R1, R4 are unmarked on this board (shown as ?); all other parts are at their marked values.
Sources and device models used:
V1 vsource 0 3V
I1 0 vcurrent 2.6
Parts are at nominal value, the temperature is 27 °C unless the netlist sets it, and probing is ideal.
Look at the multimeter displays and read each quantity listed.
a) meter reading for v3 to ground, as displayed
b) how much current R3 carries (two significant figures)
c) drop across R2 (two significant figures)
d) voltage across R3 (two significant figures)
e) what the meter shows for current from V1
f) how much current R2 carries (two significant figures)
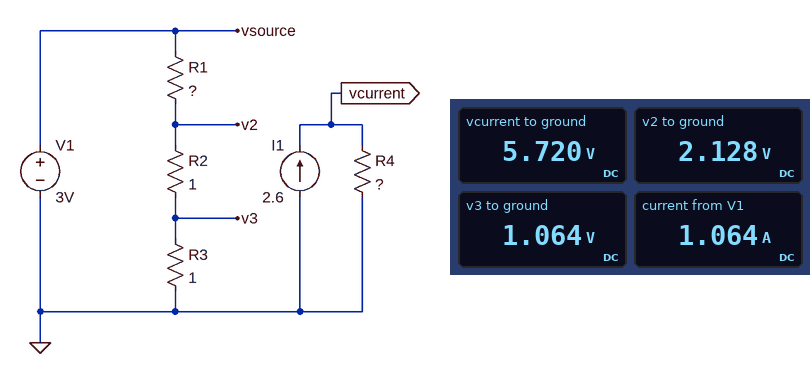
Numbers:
1.064 V
1.1 A
1.1 V
1.1 V
1.064 A
1.1 A
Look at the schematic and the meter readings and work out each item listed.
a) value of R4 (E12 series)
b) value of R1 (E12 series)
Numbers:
2.2 Ω
0.82 Ω
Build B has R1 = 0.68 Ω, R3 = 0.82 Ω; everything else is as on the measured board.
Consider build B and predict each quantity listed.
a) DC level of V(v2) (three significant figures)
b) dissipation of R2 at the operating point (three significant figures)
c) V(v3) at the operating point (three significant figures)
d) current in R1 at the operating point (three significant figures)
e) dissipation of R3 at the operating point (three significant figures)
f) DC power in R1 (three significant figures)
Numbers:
2.18 V
1.44 W
984 mV
1.20 A
1.18 W
979 mW
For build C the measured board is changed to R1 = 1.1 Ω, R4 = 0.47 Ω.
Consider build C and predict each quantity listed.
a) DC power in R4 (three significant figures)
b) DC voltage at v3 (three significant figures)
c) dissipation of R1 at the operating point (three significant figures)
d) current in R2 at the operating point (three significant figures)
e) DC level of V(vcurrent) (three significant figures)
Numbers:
3.18 W
968 mV
1.03 W
968 mA
1.22 V
